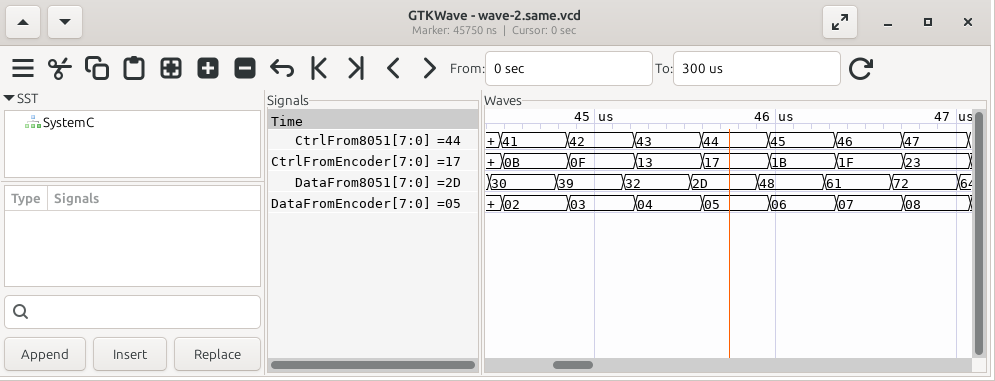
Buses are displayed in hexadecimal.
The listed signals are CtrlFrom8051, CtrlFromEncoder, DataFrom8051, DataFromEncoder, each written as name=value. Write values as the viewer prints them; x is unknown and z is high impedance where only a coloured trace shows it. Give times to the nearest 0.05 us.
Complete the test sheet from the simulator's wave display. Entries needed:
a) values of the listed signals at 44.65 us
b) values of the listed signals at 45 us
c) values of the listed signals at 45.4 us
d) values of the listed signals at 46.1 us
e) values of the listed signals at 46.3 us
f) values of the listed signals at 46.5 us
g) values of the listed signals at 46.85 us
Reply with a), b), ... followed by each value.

a) CtrlFrom8051=41, CtrlFromEncoder=0B, DataFrom8051=30, DataFromEncoder=02
b) CtrlFrom8051=42, CtrlFromEncoder=0F, DataFrom8051=39, DataFromEncoder=03
c) CtrlFrom8051=43, CtrlFromEncoder=13, DataFrom8051=32, DataFromEncoder=04
d) CtrlFrom8051=45, CtrlFromEncoder=1B, DataFrom8051=48, DataFromEncoder=06
e) CtrlFrom8051=45, CtrlFromEncoder=1B, DataFrom8051=61, DataFromEncoder=06
f) CtrlFrom8051=46, CtrlFromEncoder=1F, DataFrom8051=61, DataFromEncoder=07
g) CtrlFrom8051=47, CtrlFromEncoder=23, DataFrom8051=72, DataFromEncoder=08
